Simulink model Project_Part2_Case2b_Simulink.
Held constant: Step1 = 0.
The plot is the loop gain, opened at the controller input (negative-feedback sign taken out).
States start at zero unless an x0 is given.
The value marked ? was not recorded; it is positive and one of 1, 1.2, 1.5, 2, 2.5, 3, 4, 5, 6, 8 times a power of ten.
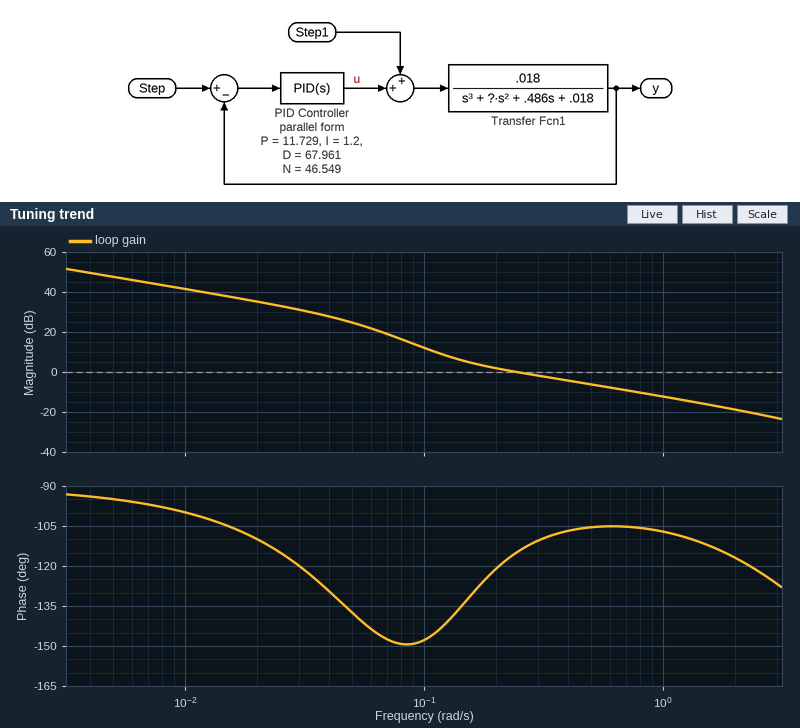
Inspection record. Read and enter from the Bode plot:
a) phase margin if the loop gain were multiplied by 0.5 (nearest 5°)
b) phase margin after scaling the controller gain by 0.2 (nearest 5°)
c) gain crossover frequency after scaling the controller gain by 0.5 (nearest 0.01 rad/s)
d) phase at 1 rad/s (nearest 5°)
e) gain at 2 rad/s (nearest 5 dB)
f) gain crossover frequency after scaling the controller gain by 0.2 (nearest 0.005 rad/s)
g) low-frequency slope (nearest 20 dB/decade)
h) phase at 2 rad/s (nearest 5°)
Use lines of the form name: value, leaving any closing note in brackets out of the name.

phase margin if the loop gain were multiplied by 0.5: 45°
phase margin after scaling the controller gain by 0.2: 30°
gain crossover frequency after scaling the controller gain by 0.5: 0.14 rad/s
phase at 1 rad/s: -105°
gain at 2 rad/s: -20 dB
gain crossover frequency after scaling the controller gain by 0.2: 0.090 rad/s
low-frequency slope: -20 dB/decade
phase at 2 rad/s: -115°
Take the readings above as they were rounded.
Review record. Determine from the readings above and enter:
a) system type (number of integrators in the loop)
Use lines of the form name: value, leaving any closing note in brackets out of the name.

system type: 1
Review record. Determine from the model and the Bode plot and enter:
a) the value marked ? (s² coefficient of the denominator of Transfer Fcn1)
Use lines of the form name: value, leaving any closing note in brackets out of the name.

the value marked ?: 5
